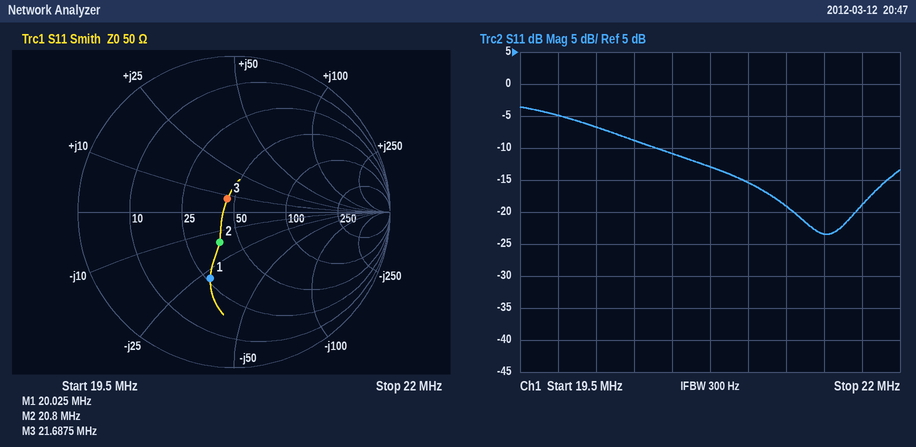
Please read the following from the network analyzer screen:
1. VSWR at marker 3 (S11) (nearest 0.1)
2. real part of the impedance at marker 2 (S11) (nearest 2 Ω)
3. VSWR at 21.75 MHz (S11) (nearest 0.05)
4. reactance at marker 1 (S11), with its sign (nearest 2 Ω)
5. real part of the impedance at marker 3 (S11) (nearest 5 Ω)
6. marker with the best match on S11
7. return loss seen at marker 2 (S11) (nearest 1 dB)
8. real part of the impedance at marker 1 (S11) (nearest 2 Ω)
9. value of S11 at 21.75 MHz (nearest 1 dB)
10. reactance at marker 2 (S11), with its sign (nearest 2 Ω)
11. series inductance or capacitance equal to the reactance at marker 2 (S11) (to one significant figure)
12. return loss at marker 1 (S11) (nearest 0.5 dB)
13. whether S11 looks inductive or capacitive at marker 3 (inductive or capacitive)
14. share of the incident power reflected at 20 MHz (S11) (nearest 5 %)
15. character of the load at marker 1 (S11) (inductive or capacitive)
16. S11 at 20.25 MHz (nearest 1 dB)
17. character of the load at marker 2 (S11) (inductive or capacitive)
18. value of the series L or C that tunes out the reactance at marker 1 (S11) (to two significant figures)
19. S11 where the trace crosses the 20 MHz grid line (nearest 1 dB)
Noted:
1.2
38 Ω
1.25
-28 Ω
45 Ω
marker 3
13 dB
26 Ω
-19 dB
-16 Ω
500 pF
7.0 dB
inductive
20 %
capacitive
-9 dB
capacitive
220 nH
-7 dB
